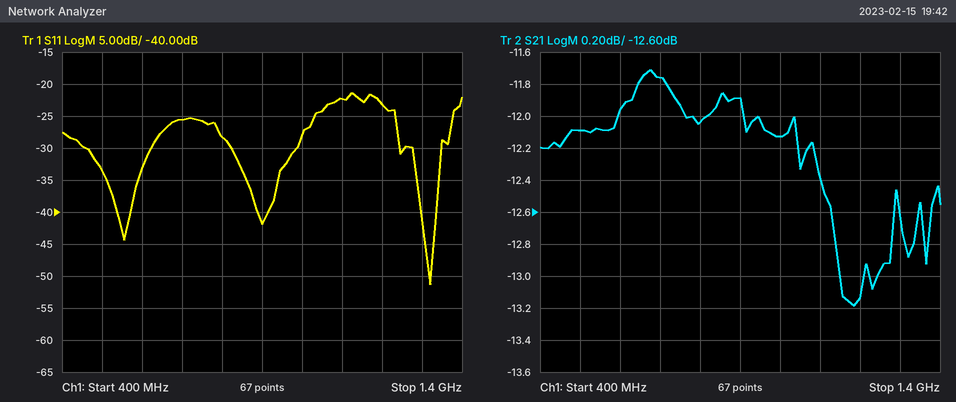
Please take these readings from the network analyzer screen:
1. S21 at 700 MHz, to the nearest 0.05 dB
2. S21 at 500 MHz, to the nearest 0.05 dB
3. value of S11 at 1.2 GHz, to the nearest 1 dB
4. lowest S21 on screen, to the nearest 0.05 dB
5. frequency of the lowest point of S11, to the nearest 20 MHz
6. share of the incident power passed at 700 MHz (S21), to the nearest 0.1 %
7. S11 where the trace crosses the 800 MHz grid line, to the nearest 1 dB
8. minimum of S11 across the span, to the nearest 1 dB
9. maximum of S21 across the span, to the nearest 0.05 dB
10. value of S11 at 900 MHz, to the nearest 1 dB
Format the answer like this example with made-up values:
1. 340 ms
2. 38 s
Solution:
1. -11.75 dB
2. -12.10 dB
3. -23 dB
4. -13.20 dB
5. 1.32 GHz
6. 6.7 %
7. -28 dB
8. -51 dB
9. -11.70 dB
10. -42 dB
